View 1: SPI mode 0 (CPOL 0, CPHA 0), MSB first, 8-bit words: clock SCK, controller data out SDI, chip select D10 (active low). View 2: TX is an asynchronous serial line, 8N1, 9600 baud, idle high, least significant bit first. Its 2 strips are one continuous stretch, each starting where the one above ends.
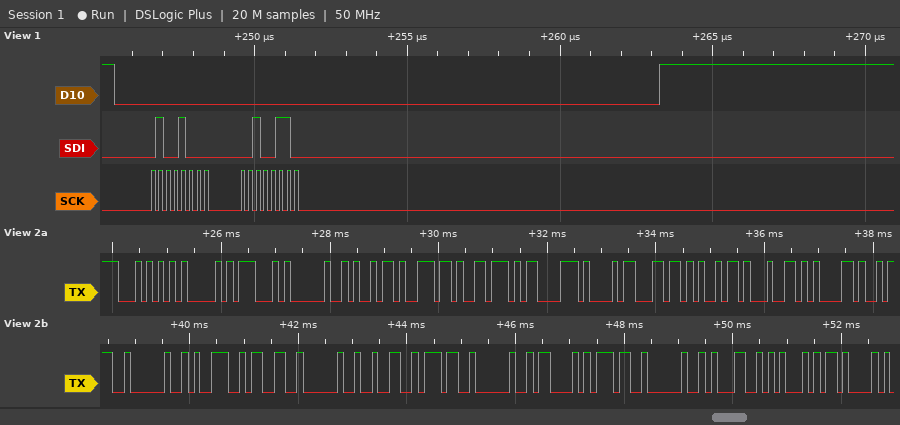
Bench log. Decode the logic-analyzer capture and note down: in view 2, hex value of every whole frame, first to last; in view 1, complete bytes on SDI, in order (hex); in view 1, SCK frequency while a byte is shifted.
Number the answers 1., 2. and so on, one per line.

1. 0x54 0x41 0x47 0x20 0x69 0x6E 0x76 0xC3 0xA1 0x6C 0x69 0x64 0x61 0x3A 0x20 0x39 0x33 0x20 0x32 0x37 0x20 0x43 0x37 0x20 0x31 0x45 0x0B
2. 0x48 0x26
3. 4 MHz
